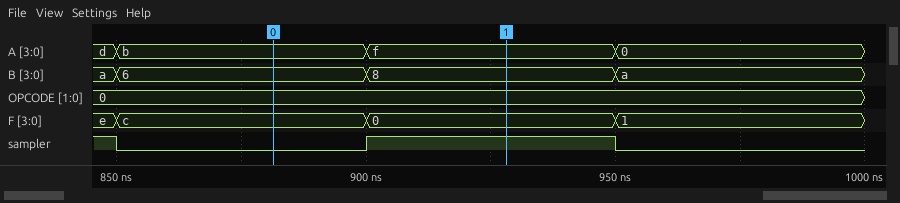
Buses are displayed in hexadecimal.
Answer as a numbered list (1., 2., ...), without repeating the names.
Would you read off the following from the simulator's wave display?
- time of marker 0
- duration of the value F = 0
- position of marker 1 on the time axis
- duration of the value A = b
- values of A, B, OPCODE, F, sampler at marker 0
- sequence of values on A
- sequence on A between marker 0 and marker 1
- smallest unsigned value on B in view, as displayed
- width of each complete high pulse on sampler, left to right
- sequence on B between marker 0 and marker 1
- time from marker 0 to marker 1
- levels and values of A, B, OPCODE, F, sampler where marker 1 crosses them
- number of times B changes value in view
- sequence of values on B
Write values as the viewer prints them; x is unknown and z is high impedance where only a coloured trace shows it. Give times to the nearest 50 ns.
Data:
1. 900 ns
2. 50 ns
3. 950 ns
4. 50 ns
5. A=b, B=6, OPCODE=0, F=c, sampler=0
6. d, b, f, 0
7. b, f
8. 6
9. 50 ns
10. 6, 8
11. 50 ns
12. A=f, B=8, OPCODE=0, F=0, sampler=1
13. 3
14. a, 6, 8, a
